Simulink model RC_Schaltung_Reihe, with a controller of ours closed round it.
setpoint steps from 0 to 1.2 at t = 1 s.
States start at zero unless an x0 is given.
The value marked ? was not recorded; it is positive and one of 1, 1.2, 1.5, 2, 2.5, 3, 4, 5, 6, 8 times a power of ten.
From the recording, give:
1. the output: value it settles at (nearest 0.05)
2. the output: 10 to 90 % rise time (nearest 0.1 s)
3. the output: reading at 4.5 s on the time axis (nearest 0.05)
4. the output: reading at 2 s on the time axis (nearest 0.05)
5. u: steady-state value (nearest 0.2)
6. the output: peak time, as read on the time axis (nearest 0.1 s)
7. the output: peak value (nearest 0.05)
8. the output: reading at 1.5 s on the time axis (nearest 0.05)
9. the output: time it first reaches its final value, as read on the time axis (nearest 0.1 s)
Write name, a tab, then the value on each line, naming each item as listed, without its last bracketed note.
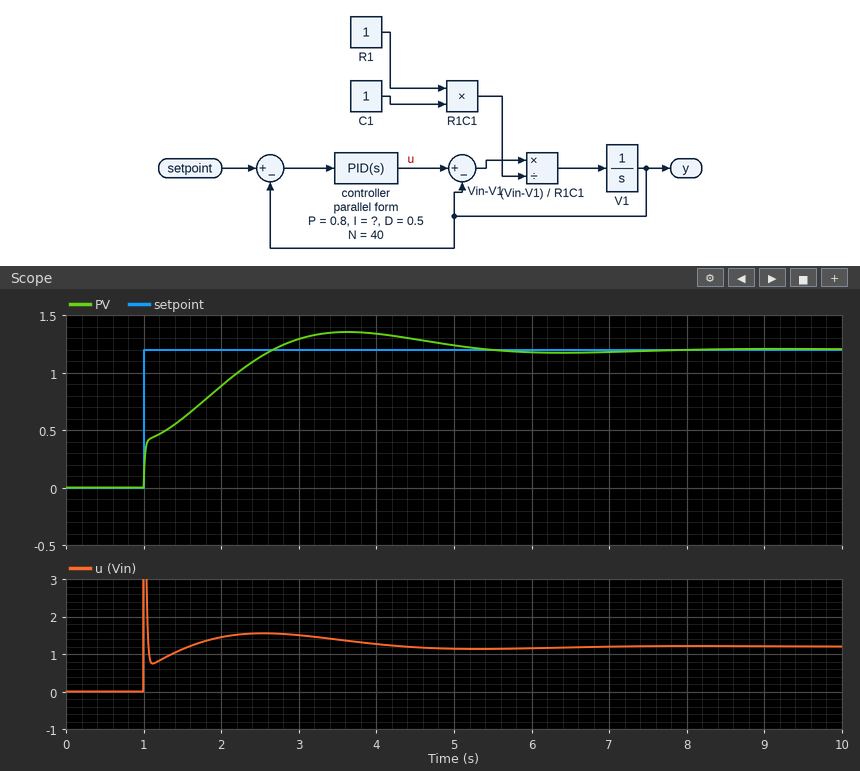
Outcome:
the output: value it settles at	1.20
the output: 10 to 90 % rise time	1.4 s
the output: reading at 4.5 s on the time axis	1.30
the output: reading at 2 s on the time axis	0.90
u: steady-state value	1.2
the output: peak time, as read on the time axis	3.6 s
the output: peak value	1.35
the output: reading at 1.5 s on the time axis	0.60
the output: time it first reaches its final value, as read on the time axis	2.7 s
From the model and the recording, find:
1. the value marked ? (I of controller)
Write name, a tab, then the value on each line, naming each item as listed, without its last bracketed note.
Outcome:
the value marked ?	2.5
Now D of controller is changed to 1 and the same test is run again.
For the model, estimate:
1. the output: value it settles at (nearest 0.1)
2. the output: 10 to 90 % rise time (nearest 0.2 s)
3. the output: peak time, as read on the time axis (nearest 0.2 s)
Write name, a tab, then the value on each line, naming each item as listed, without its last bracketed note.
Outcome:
the output: value it settles at	1.2
the output: 10 to 90 % rise time	1.6 s
the output: peak time, as read on the time axis	4.2 s
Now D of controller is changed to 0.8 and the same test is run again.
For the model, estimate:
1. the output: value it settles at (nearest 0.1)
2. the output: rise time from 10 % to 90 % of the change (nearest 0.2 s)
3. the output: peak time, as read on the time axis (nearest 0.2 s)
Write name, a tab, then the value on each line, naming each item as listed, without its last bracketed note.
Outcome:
the output: value it settles at	1.2
the output: rise time from 10 % to 90 % of the change	1.6 s
the output: peak time, as read on the time axis	4.0 s
